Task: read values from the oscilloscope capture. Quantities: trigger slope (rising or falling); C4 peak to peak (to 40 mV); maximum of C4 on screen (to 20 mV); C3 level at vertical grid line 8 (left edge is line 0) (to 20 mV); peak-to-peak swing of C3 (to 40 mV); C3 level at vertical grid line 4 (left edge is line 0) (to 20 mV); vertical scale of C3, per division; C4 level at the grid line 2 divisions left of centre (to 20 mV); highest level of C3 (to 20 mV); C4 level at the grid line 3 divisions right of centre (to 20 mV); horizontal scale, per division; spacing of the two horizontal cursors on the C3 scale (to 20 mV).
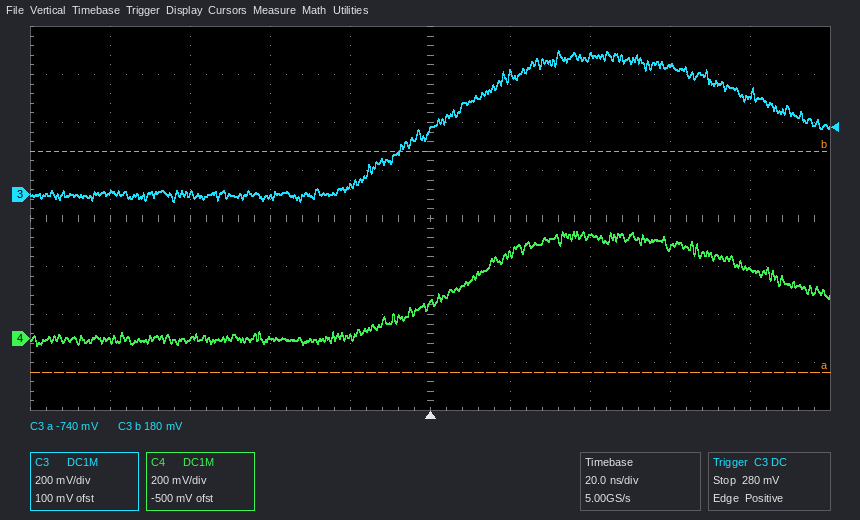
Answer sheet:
rising
480 mV
440 mV
540 mV
640 mV
40 mV
200 mV
0 mV
600 mV
380 mV
20 ns
920 mV
